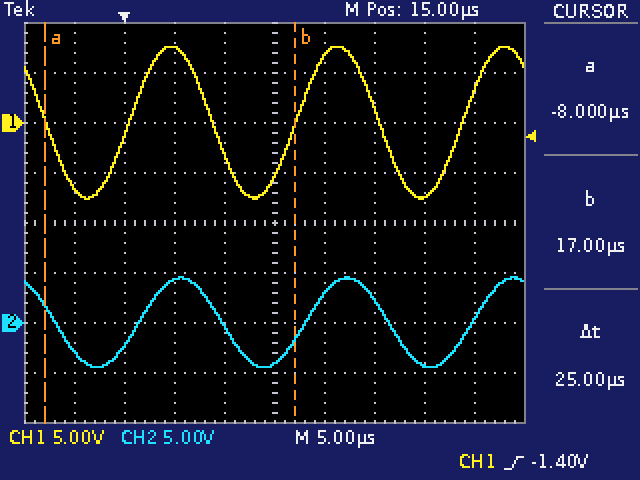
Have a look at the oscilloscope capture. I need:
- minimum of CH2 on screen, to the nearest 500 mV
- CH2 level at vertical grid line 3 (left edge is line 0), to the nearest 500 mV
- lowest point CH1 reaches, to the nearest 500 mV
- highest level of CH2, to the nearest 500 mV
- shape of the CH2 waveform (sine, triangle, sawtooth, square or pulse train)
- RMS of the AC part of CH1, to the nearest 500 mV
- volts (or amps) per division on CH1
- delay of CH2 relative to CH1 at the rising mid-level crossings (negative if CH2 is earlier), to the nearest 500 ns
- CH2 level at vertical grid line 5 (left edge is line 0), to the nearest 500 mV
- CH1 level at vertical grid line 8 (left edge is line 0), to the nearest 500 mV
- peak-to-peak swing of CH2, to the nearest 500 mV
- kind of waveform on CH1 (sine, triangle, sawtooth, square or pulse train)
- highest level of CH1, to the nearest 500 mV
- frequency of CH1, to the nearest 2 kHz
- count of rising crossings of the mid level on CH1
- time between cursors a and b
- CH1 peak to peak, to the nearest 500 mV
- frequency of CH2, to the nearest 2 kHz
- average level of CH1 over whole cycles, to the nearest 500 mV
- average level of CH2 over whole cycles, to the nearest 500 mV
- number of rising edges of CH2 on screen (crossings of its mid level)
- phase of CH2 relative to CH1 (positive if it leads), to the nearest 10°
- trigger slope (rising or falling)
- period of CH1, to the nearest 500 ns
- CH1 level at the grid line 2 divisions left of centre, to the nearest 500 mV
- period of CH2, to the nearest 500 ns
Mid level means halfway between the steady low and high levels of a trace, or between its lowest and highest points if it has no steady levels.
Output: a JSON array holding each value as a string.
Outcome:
["-4.5 V", "4.5 V", "-7.5 V", "4.5 V", "sine", "5.5 V", "5 V", "+1.0 µs", "-4.0 V", "-7.5 V", "9.0 V", "sine", "7.5 V", "60 kHz", "3", "25 µs", "15.0 V", "60 kHz", "0.0 V", "0.0 V", "3", "-20°", "rising", "16.5 µs", "7.5 V", "16.5 µs"]
